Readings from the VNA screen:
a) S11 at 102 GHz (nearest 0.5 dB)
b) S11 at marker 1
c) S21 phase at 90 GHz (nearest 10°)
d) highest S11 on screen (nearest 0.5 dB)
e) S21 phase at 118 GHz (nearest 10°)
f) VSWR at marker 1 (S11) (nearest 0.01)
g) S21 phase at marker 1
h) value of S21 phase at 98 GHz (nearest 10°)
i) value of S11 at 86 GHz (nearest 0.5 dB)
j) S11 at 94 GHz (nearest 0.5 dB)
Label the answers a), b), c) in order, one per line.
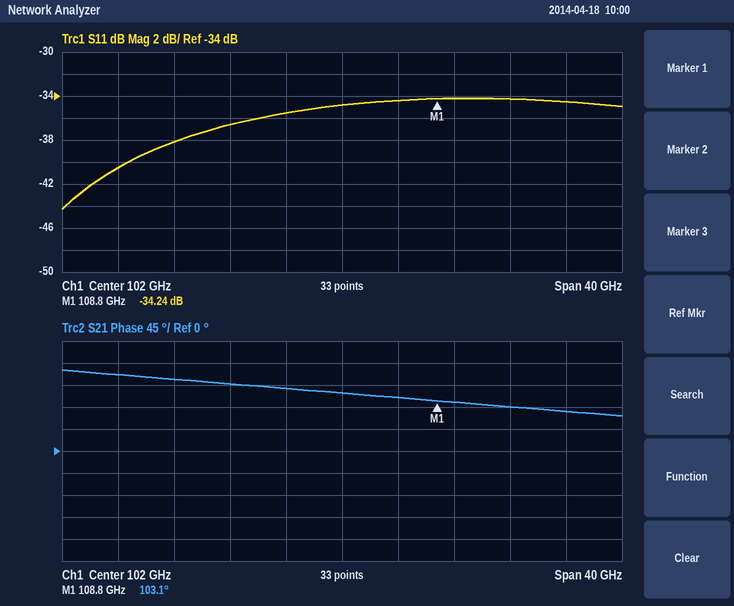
a) -35.0 dB
b) -34.24 dB
c) 150°
d) -34.0 dB
e) 80°
f) 1.04
g) 103.1°
h) 130°
i) -40.5 dB
j) -36.5 dB
